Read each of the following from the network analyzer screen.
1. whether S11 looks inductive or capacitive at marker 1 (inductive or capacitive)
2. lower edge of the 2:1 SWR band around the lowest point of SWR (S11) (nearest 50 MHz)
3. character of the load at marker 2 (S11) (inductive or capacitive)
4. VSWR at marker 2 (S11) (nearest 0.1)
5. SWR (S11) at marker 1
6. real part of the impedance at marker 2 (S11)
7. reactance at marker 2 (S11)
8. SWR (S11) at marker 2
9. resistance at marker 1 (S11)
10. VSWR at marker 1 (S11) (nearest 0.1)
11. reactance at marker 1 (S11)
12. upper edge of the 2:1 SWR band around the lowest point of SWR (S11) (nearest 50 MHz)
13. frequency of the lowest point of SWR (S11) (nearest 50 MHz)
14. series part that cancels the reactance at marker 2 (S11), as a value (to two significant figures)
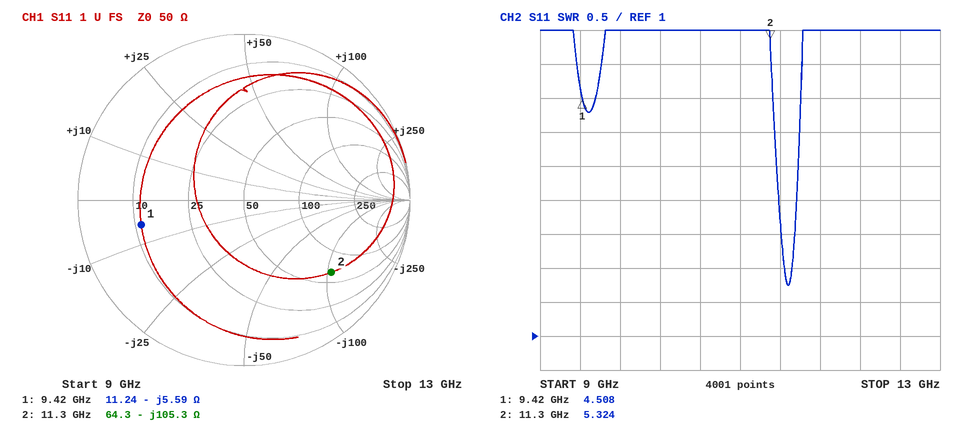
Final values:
capacitive
11.45 GHz
capacitive
5.3
4.508
64.3 Ω
-105.3 Ω
5.324
11.24 Ω
4.5
-5.59 Ω
11.50 GHz
11.50 GHz
1.5 nH
